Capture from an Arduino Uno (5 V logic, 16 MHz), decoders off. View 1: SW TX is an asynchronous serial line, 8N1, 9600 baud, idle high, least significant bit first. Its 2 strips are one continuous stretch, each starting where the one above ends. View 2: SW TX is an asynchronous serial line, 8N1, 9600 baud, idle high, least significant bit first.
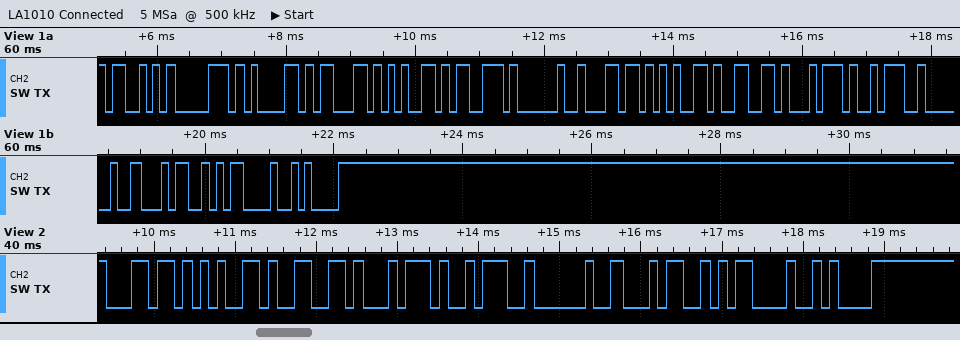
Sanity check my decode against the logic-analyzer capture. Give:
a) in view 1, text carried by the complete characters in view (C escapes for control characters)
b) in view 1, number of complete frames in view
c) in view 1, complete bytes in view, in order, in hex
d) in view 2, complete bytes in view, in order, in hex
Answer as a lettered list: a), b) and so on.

a) "Spaces left: 4\r\n"
b) 16
c) 53 70 61 63 65 73 20 6C 65 66 74 3A 20 34 0D 0A
d) 6C 65 66 74 3A 20 34 0D 0A
